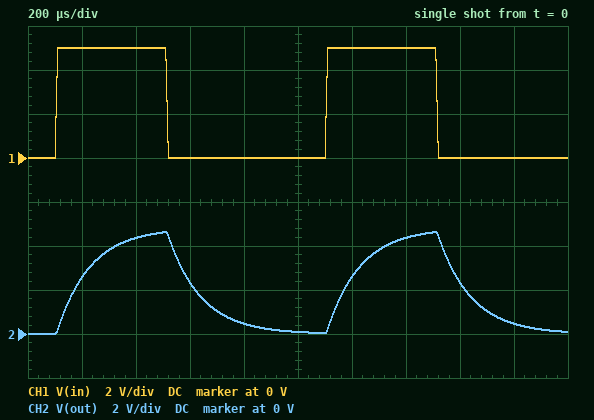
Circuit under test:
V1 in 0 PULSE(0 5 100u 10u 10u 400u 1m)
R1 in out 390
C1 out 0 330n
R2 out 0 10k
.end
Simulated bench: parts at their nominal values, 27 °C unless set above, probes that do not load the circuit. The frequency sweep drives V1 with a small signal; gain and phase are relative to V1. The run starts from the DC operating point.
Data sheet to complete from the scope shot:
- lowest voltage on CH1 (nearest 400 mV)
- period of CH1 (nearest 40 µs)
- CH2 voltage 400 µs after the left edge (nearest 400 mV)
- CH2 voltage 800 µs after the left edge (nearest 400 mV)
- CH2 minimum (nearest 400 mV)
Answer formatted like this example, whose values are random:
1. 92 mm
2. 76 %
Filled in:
1. 0 V
2. 1.00 ms
3. 4.4 V
4. 400 mV
5. 0 V
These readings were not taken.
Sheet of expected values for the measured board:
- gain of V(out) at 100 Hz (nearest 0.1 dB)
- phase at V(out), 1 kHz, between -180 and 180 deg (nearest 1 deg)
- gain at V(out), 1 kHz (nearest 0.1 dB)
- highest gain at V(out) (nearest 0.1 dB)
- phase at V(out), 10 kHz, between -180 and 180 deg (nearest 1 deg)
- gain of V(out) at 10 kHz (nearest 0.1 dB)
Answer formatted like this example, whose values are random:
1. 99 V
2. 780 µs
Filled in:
1. -0.4 dB
2. -38 deg
3. -2.4 dB
4. -0.3 dB
5. -83 deg
6. -18.2 dB
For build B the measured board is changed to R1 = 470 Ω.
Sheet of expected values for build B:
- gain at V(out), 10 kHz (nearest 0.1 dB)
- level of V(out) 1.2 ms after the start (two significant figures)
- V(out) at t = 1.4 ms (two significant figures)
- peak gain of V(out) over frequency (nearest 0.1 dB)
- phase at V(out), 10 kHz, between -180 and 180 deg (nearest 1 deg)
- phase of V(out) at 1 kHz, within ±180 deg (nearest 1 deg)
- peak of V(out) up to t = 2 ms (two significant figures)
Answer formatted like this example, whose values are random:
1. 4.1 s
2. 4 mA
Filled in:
1. -19.8 dB
2. 2.3 V
3. 4.1 V
4. -0.4 dB
5. -84 deg
6. -43 deg
7. 4.5 V
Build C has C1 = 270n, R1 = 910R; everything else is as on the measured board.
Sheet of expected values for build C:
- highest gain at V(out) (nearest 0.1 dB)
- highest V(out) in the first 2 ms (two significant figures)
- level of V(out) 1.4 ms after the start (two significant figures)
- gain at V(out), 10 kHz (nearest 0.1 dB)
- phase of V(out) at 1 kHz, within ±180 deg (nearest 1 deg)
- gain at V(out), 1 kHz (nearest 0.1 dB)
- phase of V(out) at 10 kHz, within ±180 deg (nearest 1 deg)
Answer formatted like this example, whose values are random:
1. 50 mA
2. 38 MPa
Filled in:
1. -0.8 dB
2. 3.9 V
3. 3.4 V
4. -23.8 dB
5. -55 deg
6. -5.5 dB
7. -86 deg
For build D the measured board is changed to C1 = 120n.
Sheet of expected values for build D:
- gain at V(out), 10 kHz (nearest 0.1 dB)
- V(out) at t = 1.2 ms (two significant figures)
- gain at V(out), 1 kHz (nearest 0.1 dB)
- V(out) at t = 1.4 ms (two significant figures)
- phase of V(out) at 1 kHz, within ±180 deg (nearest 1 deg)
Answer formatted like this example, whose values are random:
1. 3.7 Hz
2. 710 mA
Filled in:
1. -9.9 dB
2. 4.2 V
3. -0.7 dB
4. 4.8 V
5. -16 deg
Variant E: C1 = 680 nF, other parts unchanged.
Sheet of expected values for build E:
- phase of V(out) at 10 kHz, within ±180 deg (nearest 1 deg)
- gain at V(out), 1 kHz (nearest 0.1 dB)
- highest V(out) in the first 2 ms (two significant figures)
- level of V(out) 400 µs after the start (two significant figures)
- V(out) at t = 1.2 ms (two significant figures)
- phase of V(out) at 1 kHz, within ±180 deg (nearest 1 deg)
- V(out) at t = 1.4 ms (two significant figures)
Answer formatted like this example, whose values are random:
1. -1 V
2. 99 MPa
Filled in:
1. -86 deg
2. -5.9 dB
3. 3.9 V
4. 3.3 V
5. 1.8 V
6. -58 deg
7. 3.4 V
